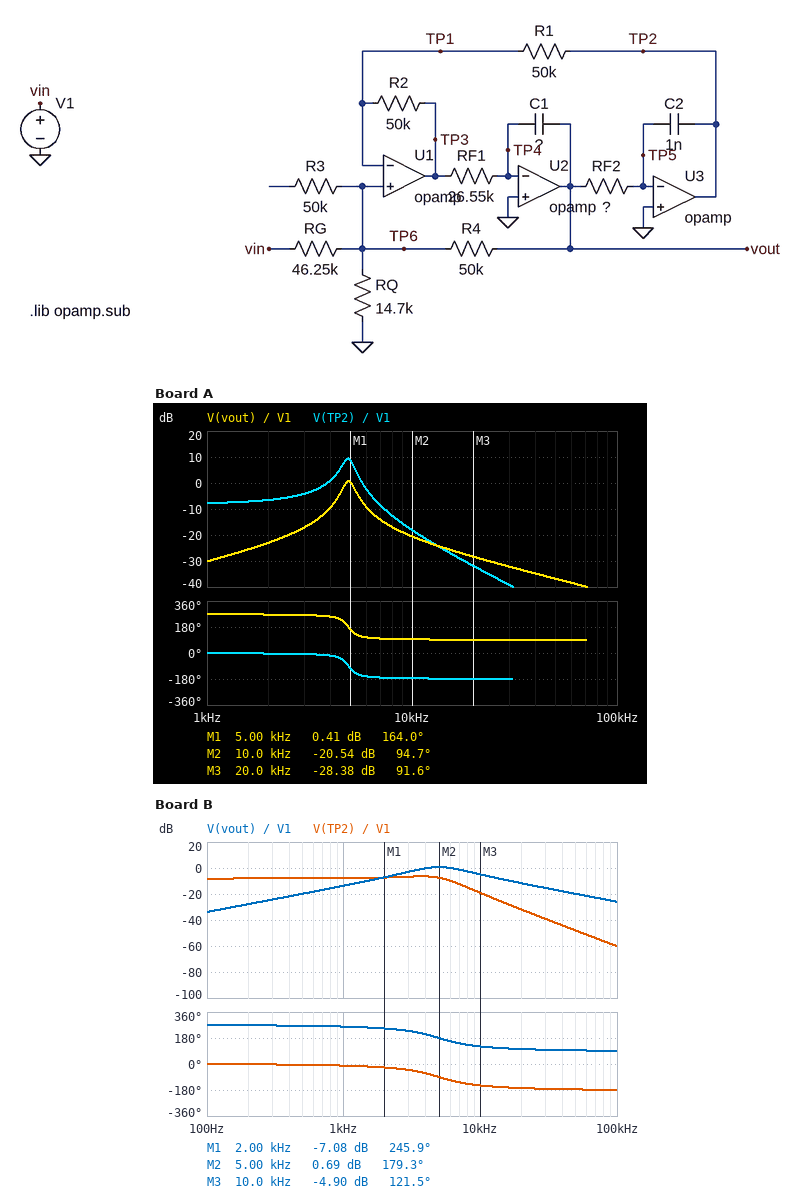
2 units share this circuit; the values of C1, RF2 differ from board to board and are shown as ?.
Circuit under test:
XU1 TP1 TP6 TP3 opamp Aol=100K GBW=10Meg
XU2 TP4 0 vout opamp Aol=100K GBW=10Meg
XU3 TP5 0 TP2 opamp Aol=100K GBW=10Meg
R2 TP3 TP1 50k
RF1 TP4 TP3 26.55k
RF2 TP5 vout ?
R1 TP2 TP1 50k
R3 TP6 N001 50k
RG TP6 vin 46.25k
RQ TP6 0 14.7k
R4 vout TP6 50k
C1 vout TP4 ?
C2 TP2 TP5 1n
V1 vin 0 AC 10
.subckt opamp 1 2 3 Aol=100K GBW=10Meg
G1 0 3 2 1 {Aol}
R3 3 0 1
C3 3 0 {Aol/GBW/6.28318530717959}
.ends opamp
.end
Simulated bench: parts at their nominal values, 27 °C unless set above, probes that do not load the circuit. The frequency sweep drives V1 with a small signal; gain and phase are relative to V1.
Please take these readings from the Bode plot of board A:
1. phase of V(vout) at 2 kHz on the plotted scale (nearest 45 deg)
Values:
270 deg
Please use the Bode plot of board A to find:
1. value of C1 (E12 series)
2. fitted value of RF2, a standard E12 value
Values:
3.3 nF
12 kΩ
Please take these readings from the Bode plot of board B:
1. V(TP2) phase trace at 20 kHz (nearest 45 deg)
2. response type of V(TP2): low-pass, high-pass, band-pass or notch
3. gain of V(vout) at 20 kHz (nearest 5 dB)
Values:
-180 deg
low-pass
-10 dB
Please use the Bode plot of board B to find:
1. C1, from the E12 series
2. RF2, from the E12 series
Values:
470 pF
82 kΩ
